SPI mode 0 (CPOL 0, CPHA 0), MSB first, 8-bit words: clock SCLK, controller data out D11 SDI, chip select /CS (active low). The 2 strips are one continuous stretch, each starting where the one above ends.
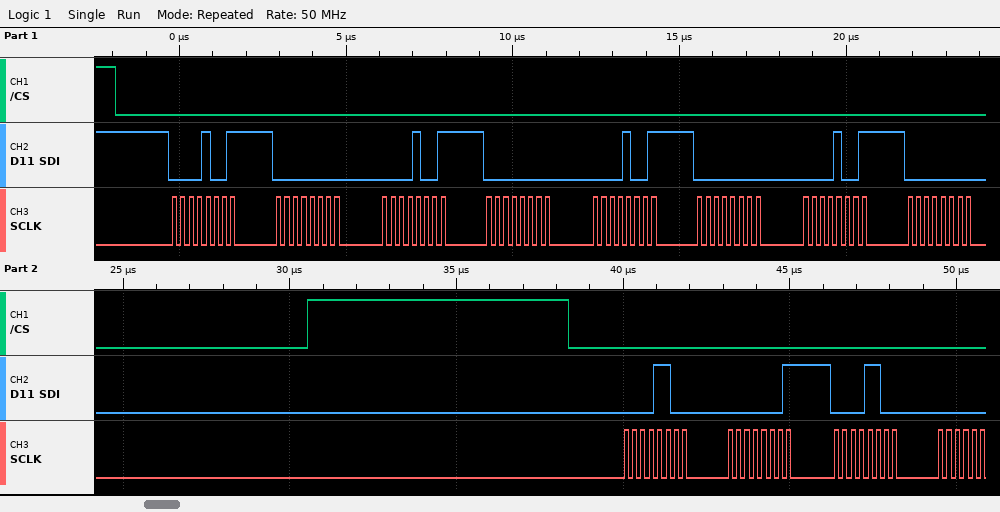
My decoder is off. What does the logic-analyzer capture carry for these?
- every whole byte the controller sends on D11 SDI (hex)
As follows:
09 00 09 00 09 00 09 00 0C 01 0C
